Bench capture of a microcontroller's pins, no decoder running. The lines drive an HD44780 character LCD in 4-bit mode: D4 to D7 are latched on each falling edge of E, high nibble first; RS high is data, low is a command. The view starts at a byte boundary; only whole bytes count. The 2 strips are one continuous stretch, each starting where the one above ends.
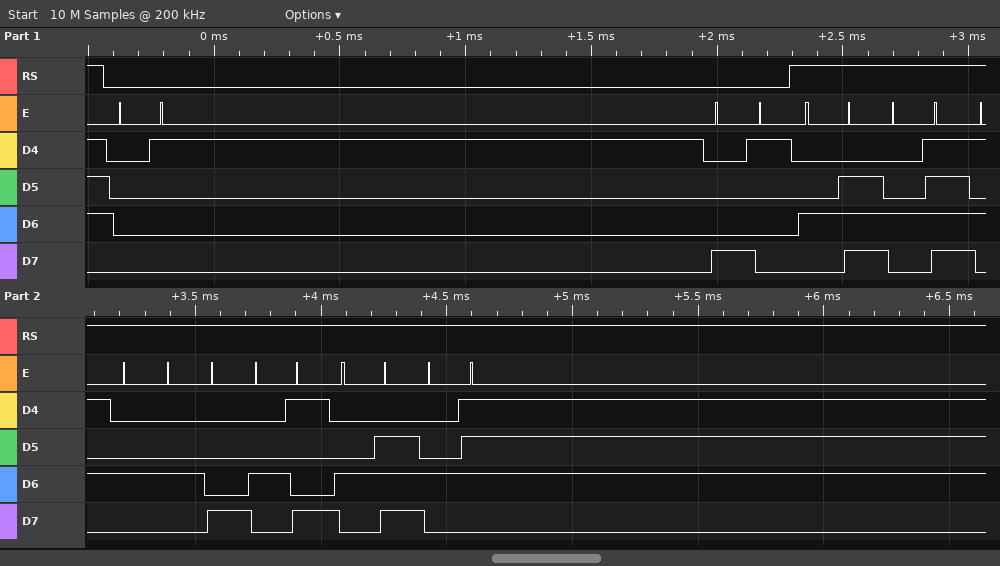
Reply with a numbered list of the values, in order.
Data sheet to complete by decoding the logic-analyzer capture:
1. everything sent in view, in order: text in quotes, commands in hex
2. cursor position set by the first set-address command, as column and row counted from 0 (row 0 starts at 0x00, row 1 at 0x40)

1. 0x01 0x81 "NOTHING"
2. column 1, row 0
